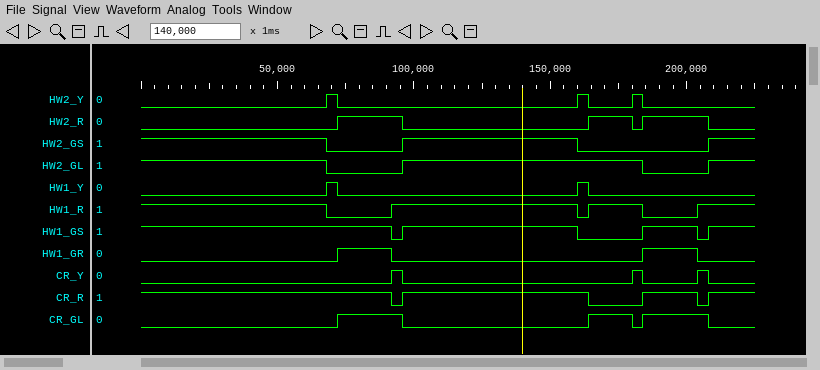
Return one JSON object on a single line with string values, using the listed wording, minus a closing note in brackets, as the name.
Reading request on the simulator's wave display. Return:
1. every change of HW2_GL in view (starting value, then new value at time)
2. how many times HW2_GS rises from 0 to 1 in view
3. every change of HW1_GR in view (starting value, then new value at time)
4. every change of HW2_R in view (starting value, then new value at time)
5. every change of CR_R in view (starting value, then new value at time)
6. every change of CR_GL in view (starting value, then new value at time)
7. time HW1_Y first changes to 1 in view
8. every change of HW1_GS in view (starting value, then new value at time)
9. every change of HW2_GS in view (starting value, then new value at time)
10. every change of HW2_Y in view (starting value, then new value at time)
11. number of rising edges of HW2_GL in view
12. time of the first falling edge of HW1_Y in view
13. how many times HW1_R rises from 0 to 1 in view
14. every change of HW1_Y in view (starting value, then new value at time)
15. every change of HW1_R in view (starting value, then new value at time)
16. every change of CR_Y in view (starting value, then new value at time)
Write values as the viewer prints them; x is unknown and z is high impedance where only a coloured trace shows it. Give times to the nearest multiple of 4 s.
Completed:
{"every change of HW2_GL in view": "1, 0 at 68 s, 1 at 96 s, 0 at 184 s, 1 at 208 s", "how many times HW2_GS rises from 0 to 1 in view": "2", "every change of HW1_GR in view": "0, 1 at 72 s, 0 at 92 s, 1 at 184 s, 0 at 204 s", "every change of HW2_R in view": "0, 1 at 72 s, 0 at 96 s, 1 at 164 s, 0 at 180 s, 1 at 184 s, 0 at 208 s", "every change of CR_R in view": "1, 0 at 92 s, 1 at 96 s, 0 at 164 s, 1 at 184 s, 0 at 204 s, 1 at 208 s", "every change of CR_GL in view": "0, 1 at 72 s, 0 at 96 s, 1 at 164 s, 0 at 180 s, 1 at 184 s, 0 at 208 s", "time HW1_Y first changes to 1 in view": "68 s", "every change of HW1_GS in view": "1, 0 at 92 s, 1 at 96 s, 0 at 160 s, 1 at 184 s, 0 at 204 s, 1 at 208 s", "every change of HW2_GS in view": "1, 0 at 68 s, 1 at 96 s, 0 at 160 s, 1 at 208 s", "every change of HW2_Y in view": "0, 1 at 68 s, 0 at 72 s, 1 at 160 s, 0 at 164 s, 1 at 180 s, 0 at 184 s", "number of rising edges of HW2_GL in view": "2", "time of the first falling edge of HW1_Y in view": "72 s", "how many times HW1_R rises from 0 to 1 in view": "3", "every change of HW1_Y in view": "0, 1 at 68 s, 0 at 72 s, 1 at 160 s, 0 at 164 s", "every change of HW1_R in view": "1, 0 at 68 s, 1 at 92 s, 0 at 160 s, 1 at 164 s, 0 at 184 s, 1 at 204 s", "every change of CR_Y in view": "0, 1 at 92 s, 0 at 96 s, 1 at 180 s, 0 at 184 s, 1 at 204 s, 0 at 208 s"}
